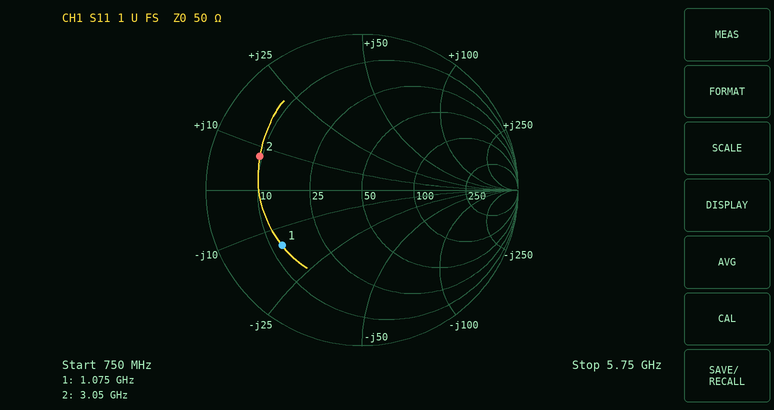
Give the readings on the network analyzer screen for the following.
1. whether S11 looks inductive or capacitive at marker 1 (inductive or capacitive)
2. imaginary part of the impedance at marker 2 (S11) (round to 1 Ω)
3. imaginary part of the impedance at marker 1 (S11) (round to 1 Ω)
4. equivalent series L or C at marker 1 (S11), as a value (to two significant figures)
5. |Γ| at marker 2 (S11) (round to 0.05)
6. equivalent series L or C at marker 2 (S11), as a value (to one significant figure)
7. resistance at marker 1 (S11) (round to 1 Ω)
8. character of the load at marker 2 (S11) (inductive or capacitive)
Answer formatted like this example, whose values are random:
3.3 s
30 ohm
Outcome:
capacitive
+8 Ω
-15 Ω
10 pF
0.70
400 pH
13 Ω
inductive
